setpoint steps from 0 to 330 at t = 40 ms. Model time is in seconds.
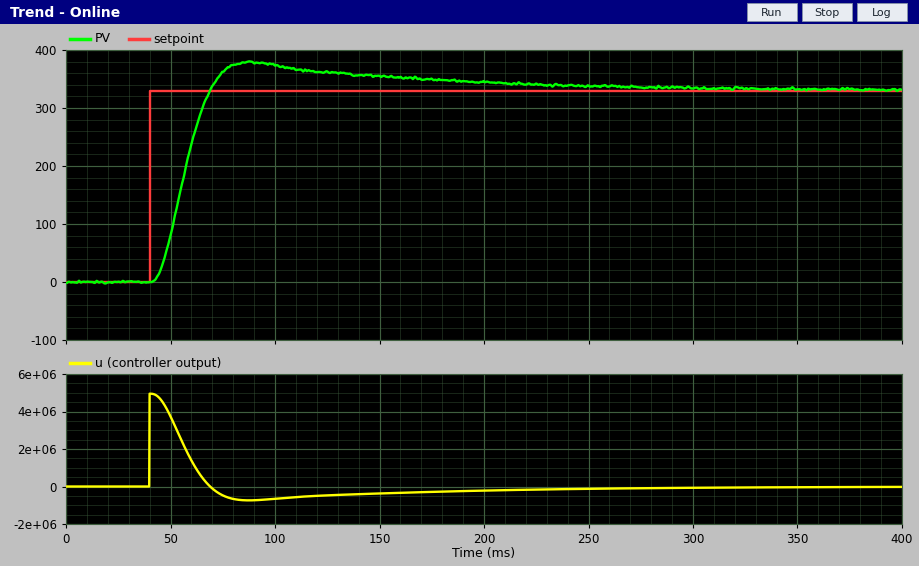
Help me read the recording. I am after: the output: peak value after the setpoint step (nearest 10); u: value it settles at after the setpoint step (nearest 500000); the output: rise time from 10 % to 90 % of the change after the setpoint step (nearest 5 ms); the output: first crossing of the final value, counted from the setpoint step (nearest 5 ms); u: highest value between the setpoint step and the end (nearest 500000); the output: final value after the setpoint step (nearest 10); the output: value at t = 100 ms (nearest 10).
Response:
380
0
20 ms
30 ms
5000000
330
370
